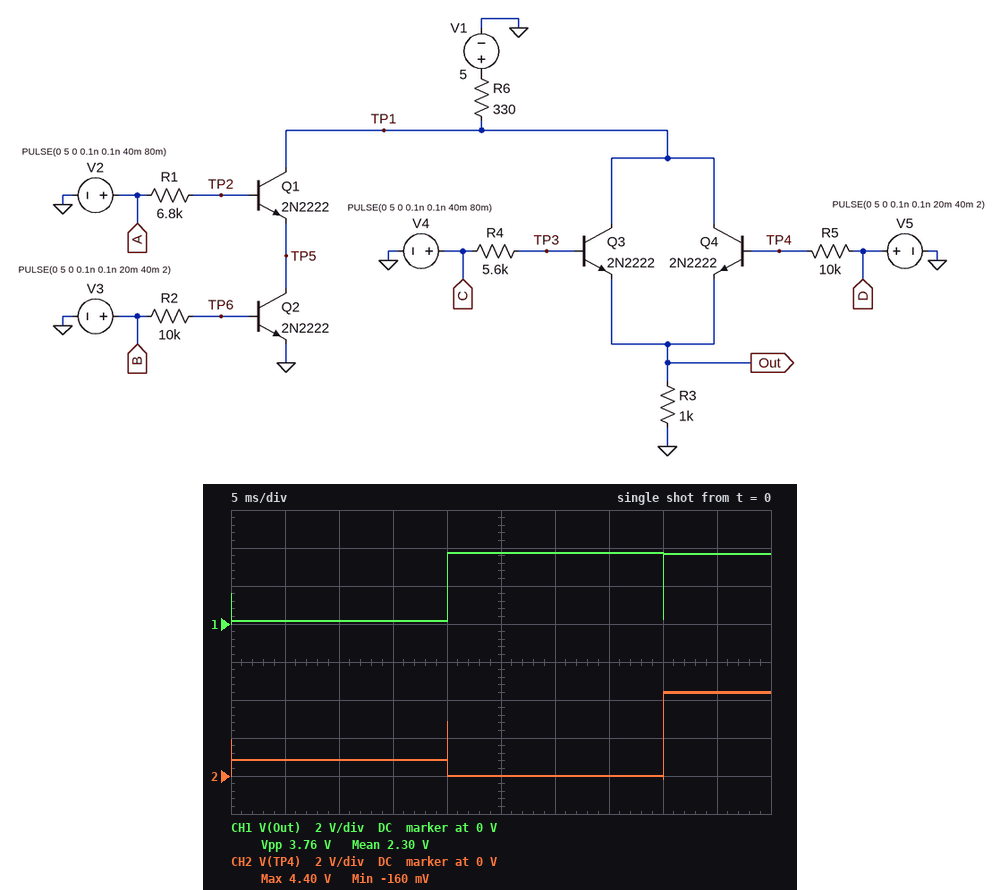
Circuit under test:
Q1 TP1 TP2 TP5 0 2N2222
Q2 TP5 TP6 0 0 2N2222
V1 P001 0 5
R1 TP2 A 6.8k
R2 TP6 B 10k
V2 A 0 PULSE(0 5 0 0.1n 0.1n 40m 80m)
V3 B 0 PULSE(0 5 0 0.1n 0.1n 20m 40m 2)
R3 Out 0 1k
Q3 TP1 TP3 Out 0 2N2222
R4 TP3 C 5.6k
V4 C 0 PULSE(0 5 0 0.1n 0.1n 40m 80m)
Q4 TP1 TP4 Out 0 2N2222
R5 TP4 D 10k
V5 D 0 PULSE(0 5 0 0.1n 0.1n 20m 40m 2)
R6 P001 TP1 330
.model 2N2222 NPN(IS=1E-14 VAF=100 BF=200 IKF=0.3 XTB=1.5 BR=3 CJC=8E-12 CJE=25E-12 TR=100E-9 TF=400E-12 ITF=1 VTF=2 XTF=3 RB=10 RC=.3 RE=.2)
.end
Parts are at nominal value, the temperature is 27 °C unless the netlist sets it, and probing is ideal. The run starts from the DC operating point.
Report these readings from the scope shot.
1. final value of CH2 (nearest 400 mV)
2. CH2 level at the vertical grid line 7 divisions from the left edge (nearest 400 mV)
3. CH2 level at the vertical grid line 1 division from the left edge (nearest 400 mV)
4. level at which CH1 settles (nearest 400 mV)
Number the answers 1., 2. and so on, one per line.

1. 4.4 V
2. 0 V
3. 800 mV
4. 3.6 V
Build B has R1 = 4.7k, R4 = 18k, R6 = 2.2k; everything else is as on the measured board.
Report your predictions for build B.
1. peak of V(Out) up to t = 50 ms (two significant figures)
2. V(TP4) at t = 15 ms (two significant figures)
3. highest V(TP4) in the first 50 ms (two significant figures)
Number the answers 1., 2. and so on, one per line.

1. 2.0 V
2. 730 mV
3. 2.4 V
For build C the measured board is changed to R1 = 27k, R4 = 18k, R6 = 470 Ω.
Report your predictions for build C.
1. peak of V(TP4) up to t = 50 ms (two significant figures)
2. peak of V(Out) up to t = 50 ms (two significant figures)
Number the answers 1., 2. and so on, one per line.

1. 4.1 V
2. 3.4 V
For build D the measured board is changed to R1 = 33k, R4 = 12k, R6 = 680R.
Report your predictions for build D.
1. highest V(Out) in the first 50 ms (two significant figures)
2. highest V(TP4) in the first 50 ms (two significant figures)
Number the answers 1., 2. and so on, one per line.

1. 3.0 V
2. 3.7 V
